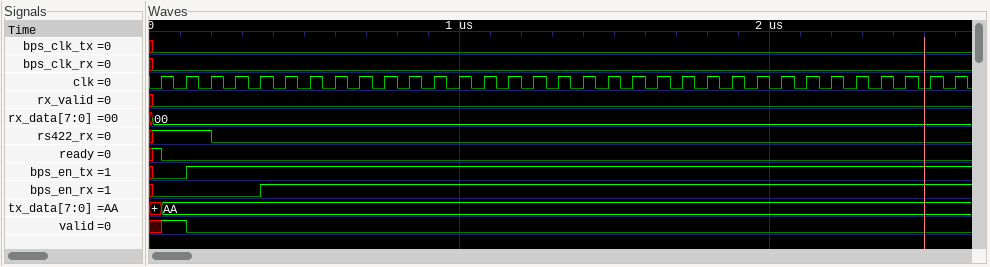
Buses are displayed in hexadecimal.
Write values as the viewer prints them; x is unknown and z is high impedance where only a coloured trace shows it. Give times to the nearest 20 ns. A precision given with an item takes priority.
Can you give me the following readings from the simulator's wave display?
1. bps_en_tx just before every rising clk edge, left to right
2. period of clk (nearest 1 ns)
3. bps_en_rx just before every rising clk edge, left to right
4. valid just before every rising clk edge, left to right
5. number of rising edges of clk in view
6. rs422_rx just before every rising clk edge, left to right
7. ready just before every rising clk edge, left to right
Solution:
0 0 1 1 1 1 1 1 1 1 1 1 1 1 1 1 1 1 1 1 1 1 1 1 1 1 1 1 1 1 1 1 1
80 ns
0 0 0 0 0 1 1 1 1 1 1 1 1 1 1 1 1 1 1 1 1 1 1 1 1 1 1 1 1 1 1 1 1
x 1 0 0 0 0 0 0 0 0 0 0 0 0 0 0 0 0 0 0 0 0 0 0 0 0 0 0 0 0 0 0 0
33
1 1 1 0 0 0 0 0 0 0 0 0 0 0 0 0 0 0 0 0 0 0 0 0 0 0 0 0 0 0 0 0 0
1 0 0 0 0 0 0 0 0 0 0 0 0 0 0 0 0 0 0 0 0 0 0 0 0 0 0 0 0 0 0 0 0
